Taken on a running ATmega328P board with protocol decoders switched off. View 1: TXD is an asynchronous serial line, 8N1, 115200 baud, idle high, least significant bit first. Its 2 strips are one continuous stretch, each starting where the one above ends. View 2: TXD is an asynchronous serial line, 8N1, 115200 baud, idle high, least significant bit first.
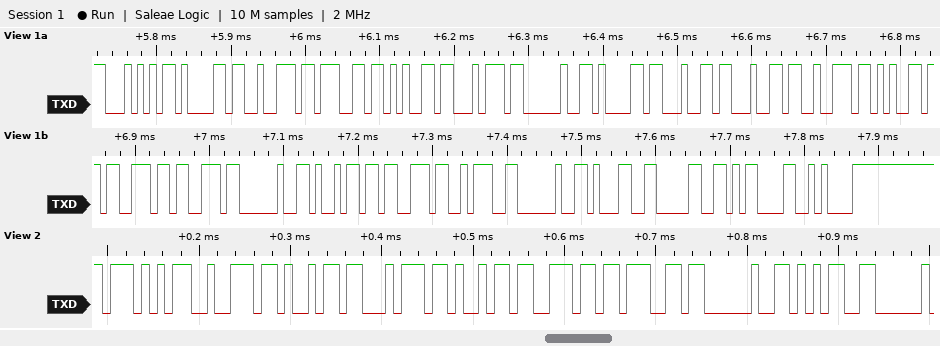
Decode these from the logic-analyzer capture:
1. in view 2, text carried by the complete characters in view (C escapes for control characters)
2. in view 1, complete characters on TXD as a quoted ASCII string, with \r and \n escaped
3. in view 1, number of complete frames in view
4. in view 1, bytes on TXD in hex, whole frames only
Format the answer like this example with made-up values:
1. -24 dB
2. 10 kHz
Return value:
1. "Writing 5"
2. "Target address is: 10\r\n"
3. 23
4. 54 61 72 67 65 74 20 61 64 64 72 65 73 73 20 69 73 3A 20 31 30 0D 0A
